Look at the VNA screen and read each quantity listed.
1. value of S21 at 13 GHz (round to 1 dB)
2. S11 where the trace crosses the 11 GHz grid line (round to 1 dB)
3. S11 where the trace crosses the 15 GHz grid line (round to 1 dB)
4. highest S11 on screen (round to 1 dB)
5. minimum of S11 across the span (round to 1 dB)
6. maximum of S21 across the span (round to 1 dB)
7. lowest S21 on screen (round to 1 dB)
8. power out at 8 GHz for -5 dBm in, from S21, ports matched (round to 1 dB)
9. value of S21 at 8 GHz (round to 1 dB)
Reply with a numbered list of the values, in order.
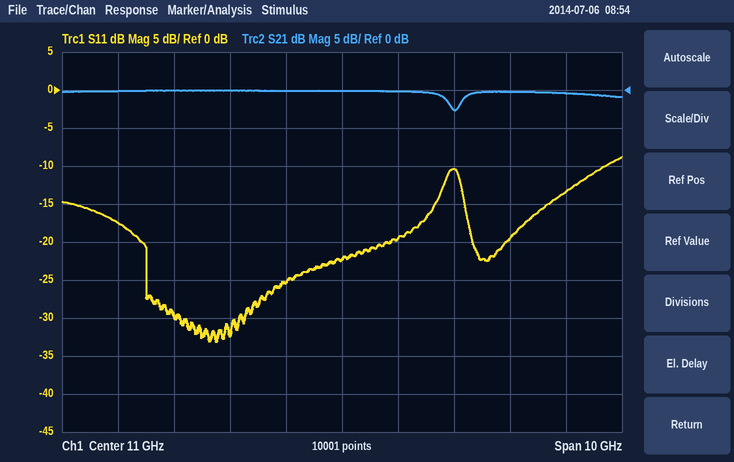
1. -3 dB
2. -22 dB
3. -13 dB
4. -9 dB
5. -33 dB
6. 0 dB
7. -3 dB
8. -5 dBm
9. 0 dB
